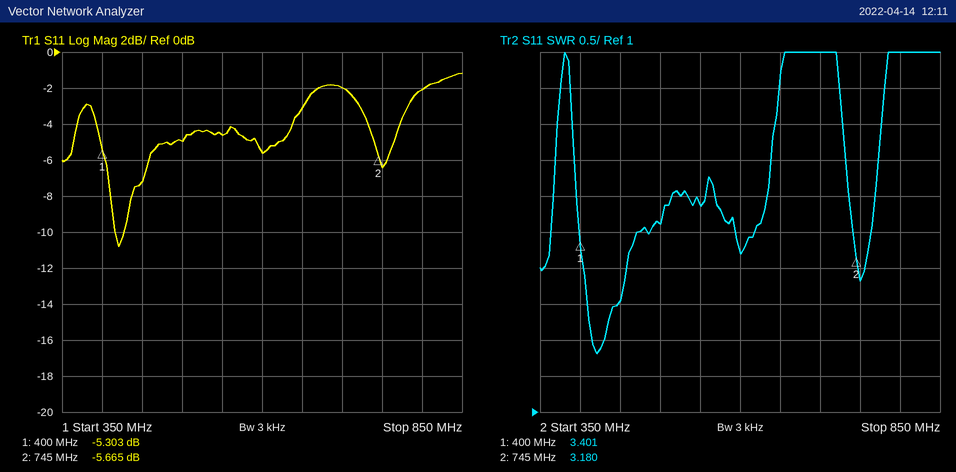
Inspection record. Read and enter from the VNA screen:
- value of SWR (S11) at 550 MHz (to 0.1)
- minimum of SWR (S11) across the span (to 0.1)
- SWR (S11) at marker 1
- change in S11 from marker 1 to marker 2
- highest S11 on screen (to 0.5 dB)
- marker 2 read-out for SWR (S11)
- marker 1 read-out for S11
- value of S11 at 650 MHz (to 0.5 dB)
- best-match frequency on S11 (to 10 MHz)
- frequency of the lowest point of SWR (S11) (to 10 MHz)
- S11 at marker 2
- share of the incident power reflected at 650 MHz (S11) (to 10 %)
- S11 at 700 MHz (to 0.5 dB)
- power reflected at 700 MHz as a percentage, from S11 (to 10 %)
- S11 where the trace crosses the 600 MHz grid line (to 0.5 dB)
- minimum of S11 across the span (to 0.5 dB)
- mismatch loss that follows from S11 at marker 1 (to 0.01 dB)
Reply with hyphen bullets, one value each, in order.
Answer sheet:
- 3.9
- 1.8
- 3.401
- -0.362 dB
- -1.0 dB
- 3.180
- -5.303 dB
- -3.0 dB
- 420 MHz
- 420 MHz
- -5.665 dB
- 50 %
- -2.0 dB
- 60 %
- -5.5 dB
- -11.0 dB
- 1.52 dB
